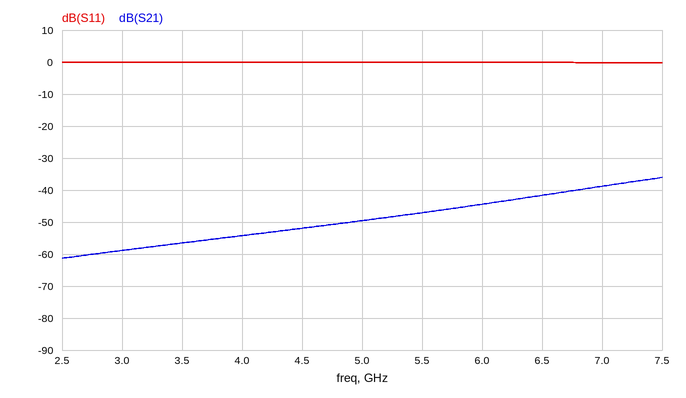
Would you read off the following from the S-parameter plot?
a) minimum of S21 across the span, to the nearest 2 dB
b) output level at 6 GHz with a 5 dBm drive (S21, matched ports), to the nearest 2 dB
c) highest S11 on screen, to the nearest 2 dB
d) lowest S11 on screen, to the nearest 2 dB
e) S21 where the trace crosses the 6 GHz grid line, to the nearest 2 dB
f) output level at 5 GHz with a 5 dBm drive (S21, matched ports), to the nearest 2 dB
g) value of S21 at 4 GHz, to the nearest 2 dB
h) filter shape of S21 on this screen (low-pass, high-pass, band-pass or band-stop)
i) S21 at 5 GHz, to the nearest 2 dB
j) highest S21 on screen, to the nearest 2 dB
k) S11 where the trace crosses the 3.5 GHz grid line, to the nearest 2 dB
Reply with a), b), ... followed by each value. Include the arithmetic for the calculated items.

a) -62 dB
b) 5 dBm + (-44 dB) = -40 dBm
c) 0 dB
d) 0 dB
e) -44 dB
f) 5 dBm + (-50 dB) = -44 dBm
g) -54 dB
h) high-pass
i) -50 dB
j) -36 dB
k) 0 dB
